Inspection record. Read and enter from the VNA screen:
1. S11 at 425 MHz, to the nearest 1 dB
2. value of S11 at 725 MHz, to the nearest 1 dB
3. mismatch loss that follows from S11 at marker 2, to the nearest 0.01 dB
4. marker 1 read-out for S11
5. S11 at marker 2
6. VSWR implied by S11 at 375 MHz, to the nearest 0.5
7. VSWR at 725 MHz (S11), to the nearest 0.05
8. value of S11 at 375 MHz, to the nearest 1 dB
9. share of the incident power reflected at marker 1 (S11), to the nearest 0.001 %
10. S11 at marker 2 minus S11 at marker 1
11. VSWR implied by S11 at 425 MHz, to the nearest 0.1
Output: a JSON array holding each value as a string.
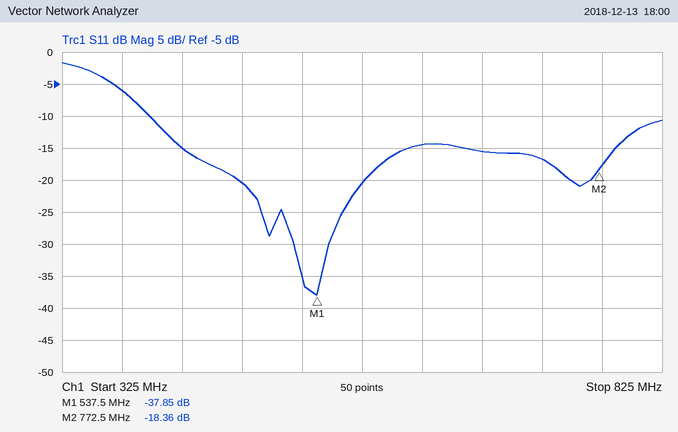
["-15 dB", "-17 dB", "0.06 dB", "-37.85 dB", "-18.36 dB", "3.0", "1.35", "-6 dB", "0.016 %", "19.49 dB", "1.4"]
